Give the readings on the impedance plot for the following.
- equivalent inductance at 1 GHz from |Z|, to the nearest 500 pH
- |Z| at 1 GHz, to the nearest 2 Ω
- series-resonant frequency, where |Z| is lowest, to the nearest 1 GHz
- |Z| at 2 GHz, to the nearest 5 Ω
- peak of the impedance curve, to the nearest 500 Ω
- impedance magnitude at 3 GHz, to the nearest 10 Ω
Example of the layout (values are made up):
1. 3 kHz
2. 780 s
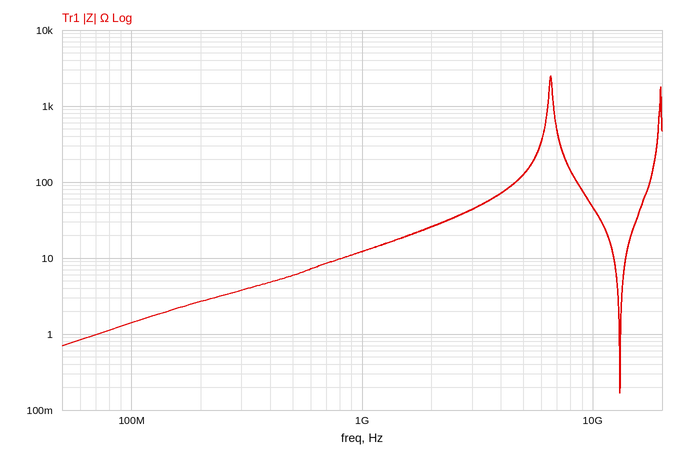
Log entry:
1. 2.0 nH
2. 12 Ω
3. 13 GHz
4. 25 Ω
5. 2.5 kΩ
6. 40 Ω
